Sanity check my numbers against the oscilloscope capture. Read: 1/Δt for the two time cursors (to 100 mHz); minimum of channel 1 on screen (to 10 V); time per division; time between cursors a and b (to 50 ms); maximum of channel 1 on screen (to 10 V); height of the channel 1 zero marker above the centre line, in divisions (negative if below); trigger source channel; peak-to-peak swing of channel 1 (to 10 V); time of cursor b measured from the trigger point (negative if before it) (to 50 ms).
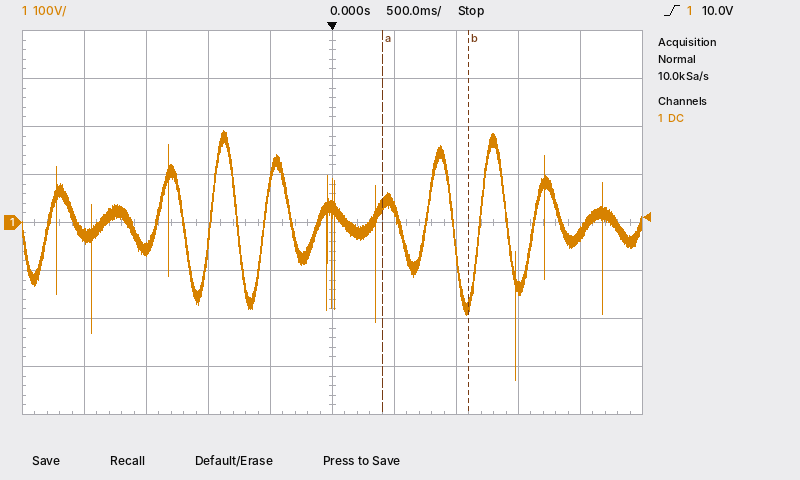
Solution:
1.4 Hz
-330 V
500 ms
700 ms
190 V
0.0 div
channel 1
520 V
+1.10 s
